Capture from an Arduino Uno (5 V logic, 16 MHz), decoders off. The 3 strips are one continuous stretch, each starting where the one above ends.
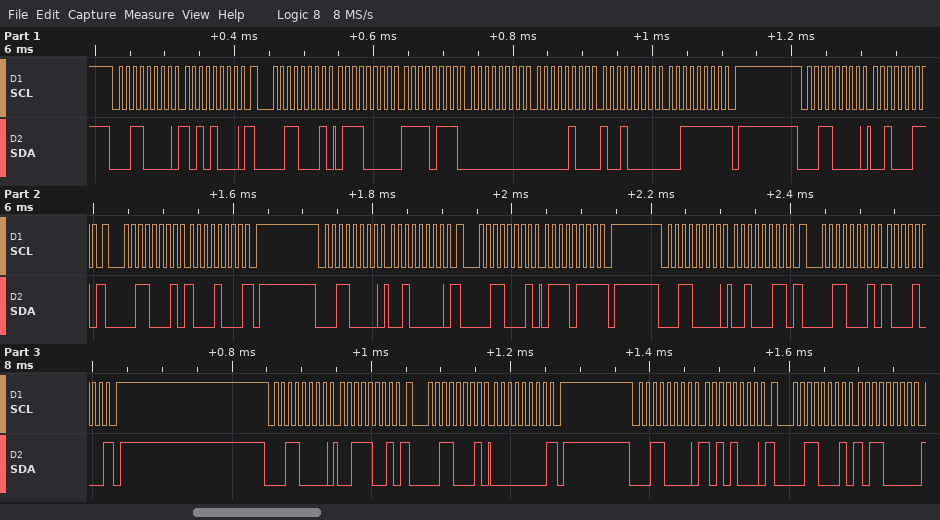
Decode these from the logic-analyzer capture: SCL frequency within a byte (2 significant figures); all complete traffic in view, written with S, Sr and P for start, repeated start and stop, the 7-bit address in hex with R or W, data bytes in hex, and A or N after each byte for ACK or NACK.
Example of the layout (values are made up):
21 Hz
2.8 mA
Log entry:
100 kHz
S 18W A A8 A Sr 18R A 70 A F7 A 00 A 04 A 90 A 3F N P S 18W A 23 A Sr 18R A 88 N P S 18W A 20 A Sr 18R A 77 N P S 18W A 23 A Sr 18R A 88 N P S 18W A 39 A Sr 18R A 00 N P S 18W A A8 A Sr 18R A B0 A
